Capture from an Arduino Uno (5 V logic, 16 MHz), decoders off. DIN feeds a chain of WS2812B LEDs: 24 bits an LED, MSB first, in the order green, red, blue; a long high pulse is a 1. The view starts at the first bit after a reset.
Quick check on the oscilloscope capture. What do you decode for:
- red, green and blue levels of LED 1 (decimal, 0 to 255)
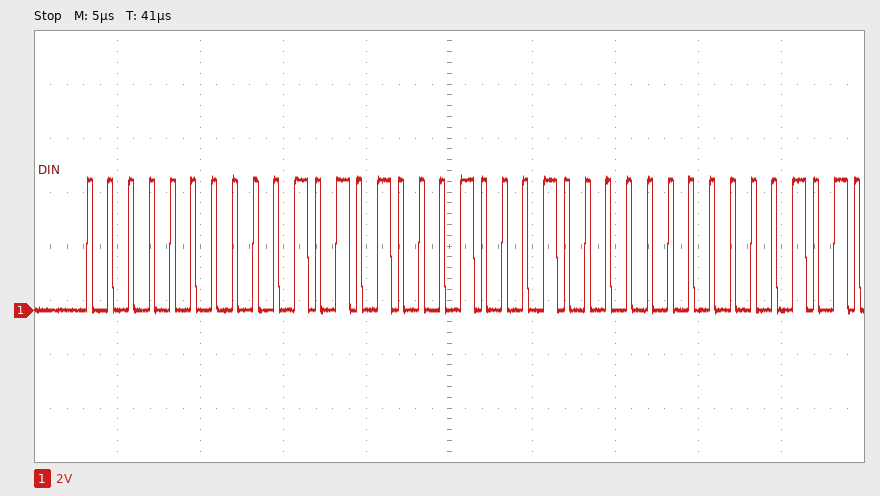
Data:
42, 0, 34
